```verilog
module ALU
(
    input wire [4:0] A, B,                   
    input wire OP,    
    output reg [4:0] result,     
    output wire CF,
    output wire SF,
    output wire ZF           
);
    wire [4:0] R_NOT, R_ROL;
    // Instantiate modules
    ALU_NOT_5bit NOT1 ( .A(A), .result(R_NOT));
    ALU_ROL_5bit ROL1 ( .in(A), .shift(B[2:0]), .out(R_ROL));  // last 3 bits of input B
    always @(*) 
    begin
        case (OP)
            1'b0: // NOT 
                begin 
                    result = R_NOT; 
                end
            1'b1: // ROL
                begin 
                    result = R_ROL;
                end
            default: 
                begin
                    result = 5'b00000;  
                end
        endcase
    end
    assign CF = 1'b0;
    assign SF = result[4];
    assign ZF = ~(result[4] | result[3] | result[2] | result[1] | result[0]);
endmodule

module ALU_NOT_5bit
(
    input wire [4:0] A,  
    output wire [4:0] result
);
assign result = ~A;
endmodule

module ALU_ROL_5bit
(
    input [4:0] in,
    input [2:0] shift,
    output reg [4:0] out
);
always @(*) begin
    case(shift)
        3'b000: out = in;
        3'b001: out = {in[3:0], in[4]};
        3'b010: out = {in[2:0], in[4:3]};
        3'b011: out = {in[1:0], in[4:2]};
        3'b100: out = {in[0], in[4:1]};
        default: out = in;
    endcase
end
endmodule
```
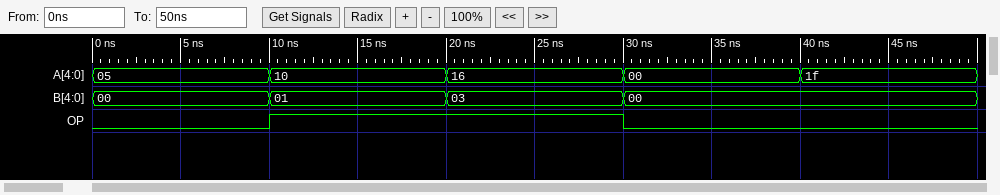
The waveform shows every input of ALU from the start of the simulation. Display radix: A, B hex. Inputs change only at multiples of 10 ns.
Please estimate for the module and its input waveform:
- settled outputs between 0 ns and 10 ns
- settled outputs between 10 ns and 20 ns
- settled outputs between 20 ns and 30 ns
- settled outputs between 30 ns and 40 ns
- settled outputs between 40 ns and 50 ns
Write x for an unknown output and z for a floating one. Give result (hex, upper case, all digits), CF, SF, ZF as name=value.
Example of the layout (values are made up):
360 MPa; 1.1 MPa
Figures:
result=1A, CF=0, SF=1, ZF=0; result=01, CF=0, SF=0, ZF=0; result=15, CF=0, SF=1, ZF=0; result=1F, CF=0, SF=1, ZF=0; result=00, CF=0, SF=0, ZF=1
